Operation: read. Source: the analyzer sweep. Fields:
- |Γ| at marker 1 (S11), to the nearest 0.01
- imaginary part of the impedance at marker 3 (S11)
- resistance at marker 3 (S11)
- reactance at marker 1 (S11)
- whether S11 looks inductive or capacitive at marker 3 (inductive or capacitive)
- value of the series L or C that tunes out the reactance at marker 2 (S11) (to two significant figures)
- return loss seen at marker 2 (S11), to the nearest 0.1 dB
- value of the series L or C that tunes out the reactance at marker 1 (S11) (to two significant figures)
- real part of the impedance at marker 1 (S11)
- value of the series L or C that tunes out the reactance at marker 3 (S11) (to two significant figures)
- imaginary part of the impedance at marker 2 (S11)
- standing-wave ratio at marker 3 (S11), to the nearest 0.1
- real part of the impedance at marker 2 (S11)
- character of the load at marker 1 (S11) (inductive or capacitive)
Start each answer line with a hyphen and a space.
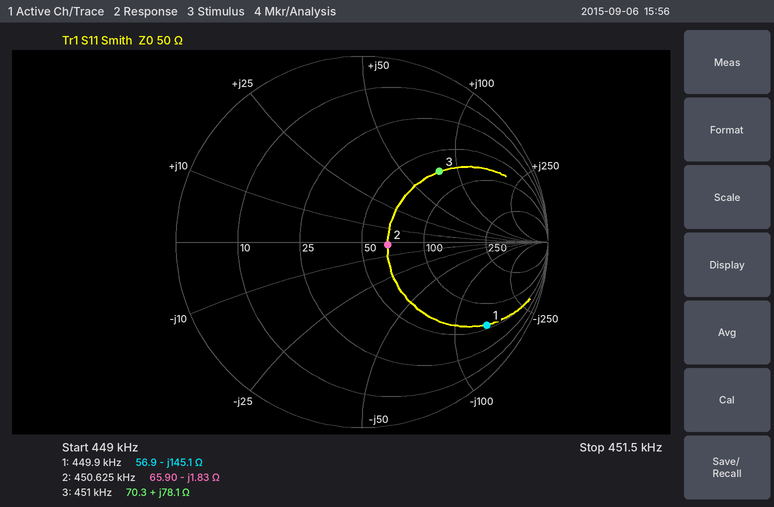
- 0.81
- +78.1 Ω
- 70.3 Ω
- -145.1 Ω
- inductive
- 650 nH
- 17.2 dB
- 51 µH
- 56.9 Ω
- 4.5 nF
- -1.83 Ω
- 3.6
- 65.90 Ω
- capacitive
